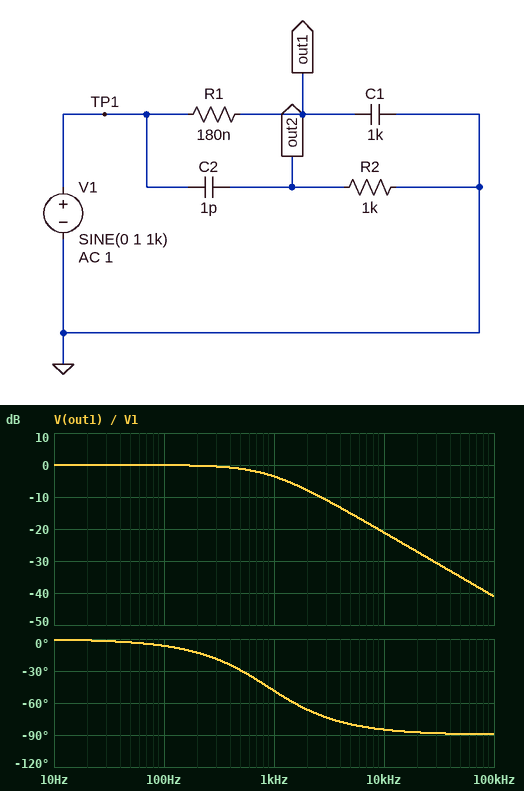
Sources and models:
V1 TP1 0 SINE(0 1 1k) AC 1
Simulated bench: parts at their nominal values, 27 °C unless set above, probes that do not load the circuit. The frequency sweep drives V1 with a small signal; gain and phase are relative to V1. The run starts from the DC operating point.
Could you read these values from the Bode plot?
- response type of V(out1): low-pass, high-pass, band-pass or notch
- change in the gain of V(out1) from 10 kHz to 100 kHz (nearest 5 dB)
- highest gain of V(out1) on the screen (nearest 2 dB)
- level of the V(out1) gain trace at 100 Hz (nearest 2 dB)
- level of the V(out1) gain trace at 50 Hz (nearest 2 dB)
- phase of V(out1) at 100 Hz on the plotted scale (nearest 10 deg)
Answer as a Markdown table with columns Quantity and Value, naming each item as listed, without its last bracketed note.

| Quantity | Value |
|---|---|
| response type of V(out1): low-pass, high-pass, band-pass or notch | low-pass |
| change in the gain of V(out1) from 10 kHz to 100 kHz | -20 dB |
| highest gain of V(out1) on the screen | 0 dB |
| level of the V(out1) gain trace at 100 Hz | 0 dB |
| level of the V(out1) gain trace at 50 Hz | 0 dB |
| phase of V(out1) at 100 Hz on the plotted scale | -10 deg |
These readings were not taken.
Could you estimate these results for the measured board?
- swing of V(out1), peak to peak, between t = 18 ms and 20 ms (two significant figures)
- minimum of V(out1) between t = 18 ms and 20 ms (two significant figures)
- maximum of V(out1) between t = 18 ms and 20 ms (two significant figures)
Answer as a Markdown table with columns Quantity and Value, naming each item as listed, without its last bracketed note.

| Quantity | Value |
|---|---|
| swing of V(out1), peak to peak, between t = 18 ms and 20 ms | 1.3 V |
| minimum of V(out1) between t = 18 ms and 20 ms | -660 mV |
| maximum of V(out1) between t = 18 ms and 20 ms | 660 mV |
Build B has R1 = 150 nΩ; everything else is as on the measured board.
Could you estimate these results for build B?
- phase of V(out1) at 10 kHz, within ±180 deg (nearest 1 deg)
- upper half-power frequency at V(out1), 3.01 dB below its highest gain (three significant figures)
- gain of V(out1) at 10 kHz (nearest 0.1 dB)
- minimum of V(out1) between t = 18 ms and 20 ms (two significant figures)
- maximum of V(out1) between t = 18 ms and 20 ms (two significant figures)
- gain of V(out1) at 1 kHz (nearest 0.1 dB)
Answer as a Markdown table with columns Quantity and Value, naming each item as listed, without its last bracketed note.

| Quantity | Value |
|---|---|
| phase of V(out1) at 10 kHz, within ±180 deg | -84 deg |
| upper half-power frequency at V(out1), 3.01 dB below its highest gain | 1.06 kHz |
| gain of V(out1) at 10 kHz | -19.5 dB |
| minimum of V(out1) between t = 18 ms and 20 ms | -730 mV |
| maximum of V(out1) between t = 18 ms and 20 ms | 730 mV |
| gain of V(out1) at 1 kHz | -2.8 dB |
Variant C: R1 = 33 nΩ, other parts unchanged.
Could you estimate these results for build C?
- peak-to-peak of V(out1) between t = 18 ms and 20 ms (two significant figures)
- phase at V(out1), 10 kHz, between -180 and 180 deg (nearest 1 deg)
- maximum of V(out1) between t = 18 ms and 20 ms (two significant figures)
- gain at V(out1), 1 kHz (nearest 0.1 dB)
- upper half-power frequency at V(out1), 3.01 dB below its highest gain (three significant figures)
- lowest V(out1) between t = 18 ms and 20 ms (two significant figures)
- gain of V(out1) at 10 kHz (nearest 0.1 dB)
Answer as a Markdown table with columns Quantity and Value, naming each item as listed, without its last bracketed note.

| Quantity | Value |
|---|---|
| peak-to-peak of V(out1) between t = 18 ms and 20 ms | 2.0 V |
| phase at V(out1), 10 kHz, between -180 and 180 deg | -64 deg |
| maximum of V(out1) between t = 18 ms and 20 ms | 980 mV |
| gain at V(out1), 1 kHz | -0.2 dB |
| upper half-power frequency at V(out1), 3.01 dB below its highest gain | 4.82 kHz |
| lowest V(out1) between t = 18 ms and 20 ms | -980 mV |
| gain of V(out1) at 10 kHz | -7.2 dB |
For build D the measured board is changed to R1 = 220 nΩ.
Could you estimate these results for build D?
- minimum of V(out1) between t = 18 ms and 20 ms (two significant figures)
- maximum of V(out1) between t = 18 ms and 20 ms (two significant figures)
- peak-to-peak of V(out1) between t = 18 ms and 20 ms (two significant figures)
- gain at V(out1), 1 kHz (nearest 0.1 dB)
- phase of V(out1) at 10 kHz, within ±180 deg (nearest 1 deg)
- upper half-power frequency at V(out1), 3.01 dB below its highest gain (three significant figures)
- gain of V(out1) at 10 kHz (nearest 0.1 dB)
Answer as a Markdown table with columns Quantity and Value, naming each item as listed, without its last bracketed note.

| Quantity | Value |
|---|---|
| minimum of V(out1) between t = 18 ms and 20 ms | -590 mV |
| maximum of V(out1) between t = 18 ms and 20 ms | 590 mV |
| peak-to-peak of V(out1) between t = 18 ms and 20 ms | 1.2 V |
| gain at V(out1), 1 kHz | -4.6 dB |
| phase of V(out1) at 10 kHz, within ±180 deg | -86 deg |
| upper half-power frequency at V(out1), 3.01 dB below its highest gain | 723 Hz |
| gain of V(out1) at 10 kHz | -22.8 dB |
